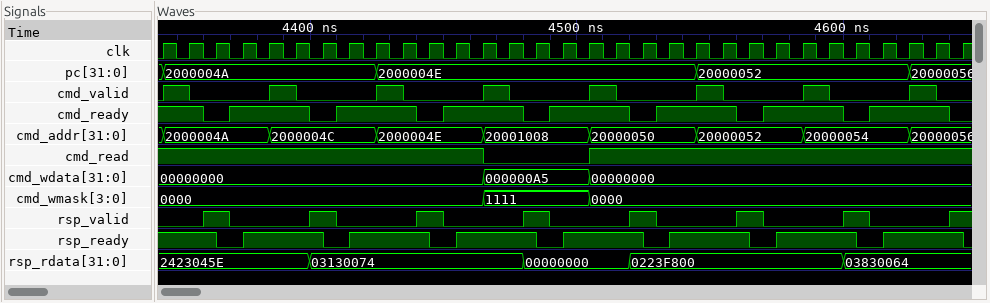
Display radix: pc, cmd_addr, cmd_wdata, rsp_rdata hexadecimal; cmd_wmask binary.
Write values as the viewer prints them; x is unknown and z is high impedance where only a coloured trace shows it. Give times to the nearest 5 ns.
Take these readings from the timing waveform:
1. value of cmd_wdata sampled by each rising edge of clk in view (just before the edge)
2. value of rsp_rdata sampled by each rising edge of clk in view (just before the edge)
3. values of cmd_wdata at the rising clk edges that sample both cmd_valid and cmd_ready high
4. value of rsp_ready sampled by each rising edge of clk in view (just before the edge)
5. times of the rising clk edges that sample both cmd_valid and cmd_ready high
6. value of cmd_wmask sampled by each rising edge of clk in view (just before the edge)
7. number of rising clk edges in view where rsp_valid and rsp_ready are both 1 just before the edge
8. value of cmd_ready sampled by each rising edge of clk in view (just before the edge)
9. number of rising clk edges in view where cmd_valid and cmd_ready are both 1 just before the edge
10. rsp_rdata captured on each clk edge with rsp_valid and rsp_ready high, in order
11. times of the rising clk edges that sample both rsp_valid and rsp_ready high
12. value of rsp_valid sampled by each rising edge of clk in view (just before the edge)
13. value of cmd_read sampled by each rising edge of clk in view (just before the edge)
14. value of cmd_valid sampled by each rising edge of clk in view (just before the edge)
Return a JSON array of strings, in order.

["00000000, 00000000, 00000000, 00000000, 00000000, 00000000, 00000000, 00000000, 00000000, 00000000, 00000000, 00000000, 00000000, 000000A5, 000000A5, 000000A5, 000000A5, 00000000, 00000000, 00000000, 00000000, 00000000, 00000000, 00000000, 00000000, 00000000, 00000000, 00000000, 00000000, 00000000, 00000000", "2423045E, 2423045E, 2423045E, 2423045E, 2423045E, 2423045E, 03130074, 03130074, 03130074, 03130074, 03130074, 03130074, 03130074, 03130074, 00000000, 00000000, 00000000, 00000000, 0223F800, 0223F800, 0223F800, 0223F800, 0223F800, 0223F800, 0223F800, 0223F800, 03830064, 03830064, 03830064, 03830064, 03830064", "00000000, 00000000, 00000000, 000000A5, 00000000, 00000000, 00000000, 00000000", "1 1 1 0 1 1 1 0 1 1 1 0 1 1 1 0 1 1 1 0 1 1 1 0 1 1 1 0 1 1 1", "4355 ns, 4395 ns, 4435 ns, 4475 ns, 4515 ns, 4555 ns, 4595 ns, 4635 ns", "0000, 0000, 0000, 0000, 0000, 0000, 0000, 0000, 0000, 0000, 0000, 0000, 0000, 1111, 1111, 1111, 1111, 0000, 0000, 0000, 0000, 0000, 0000, 0000, 0000, 0000, 0000, 0000, 0000, 0000, 0000", "8", "1 1 0 1 1 1 0 1 1 1 0 1 1 1 0 1 1 1 0 1 1 1 0 1 1 1 0 1 1 1 0", "8", "2423045E, 03130074, 03130074, 00000000, 0223F800, 0223F800, 03830064, 03830064", "4365 ns, 4405 ns, 4445 ns, 4485 ns, 4525 ns, 4565 ns, 4605 ns, 4645 ns", "0 0 1 0 0 0 1 0 0 0 1 0 0 0 1 0 0 0 1 0 0 0 1 0 0 0 1 0 0 0 1", "1 1 1 1 1 1 1 1 1 1 1 1 1 0 0 0 0 1 1 1 1 1 1 1 1 1 1 1 1 1 1", "0 1 0 0 0 1 0 0 0 1 0 0 0 1 0 0 0 1 0 0 0 1 0 0 0 1 0 0 0 1 0"]
